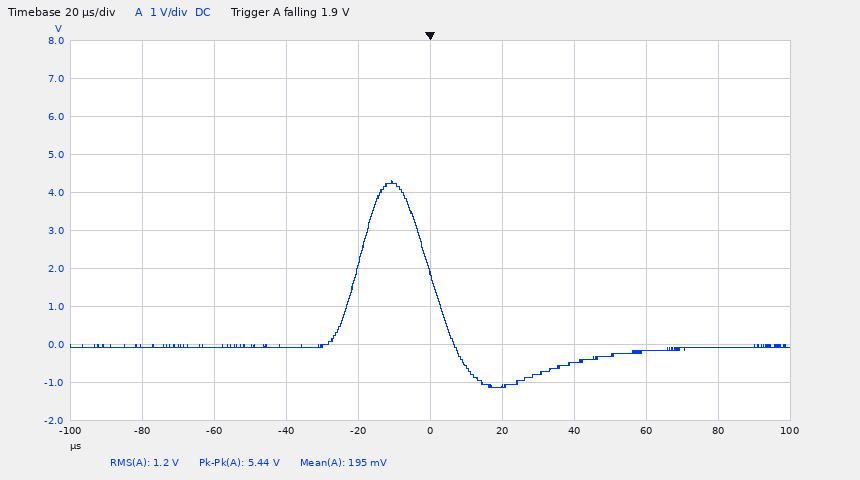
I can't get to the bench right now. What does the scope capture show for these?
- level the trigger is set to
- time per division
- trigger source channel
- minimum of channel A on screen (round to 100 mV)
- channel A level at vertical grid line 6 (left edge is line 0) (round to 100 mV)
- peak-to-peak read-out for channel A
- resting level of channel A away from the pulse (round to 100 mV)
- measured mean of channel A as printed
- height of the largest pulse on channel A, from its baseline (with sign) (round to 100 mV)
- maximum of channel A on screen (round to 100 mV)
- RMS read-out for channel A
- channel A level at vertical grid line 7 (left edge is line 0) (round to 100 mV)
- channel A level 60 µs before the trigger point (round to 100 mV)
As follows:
1.9 V
20 µs
channel A
-1.1 V
-1.1 V
5.44 V
-100 mV
195 mV
+4.4 V
4.3 V
1.2 V
-500 mV
-100 mV
